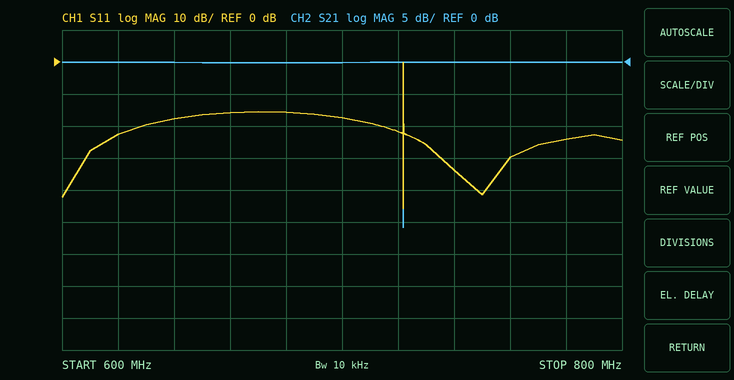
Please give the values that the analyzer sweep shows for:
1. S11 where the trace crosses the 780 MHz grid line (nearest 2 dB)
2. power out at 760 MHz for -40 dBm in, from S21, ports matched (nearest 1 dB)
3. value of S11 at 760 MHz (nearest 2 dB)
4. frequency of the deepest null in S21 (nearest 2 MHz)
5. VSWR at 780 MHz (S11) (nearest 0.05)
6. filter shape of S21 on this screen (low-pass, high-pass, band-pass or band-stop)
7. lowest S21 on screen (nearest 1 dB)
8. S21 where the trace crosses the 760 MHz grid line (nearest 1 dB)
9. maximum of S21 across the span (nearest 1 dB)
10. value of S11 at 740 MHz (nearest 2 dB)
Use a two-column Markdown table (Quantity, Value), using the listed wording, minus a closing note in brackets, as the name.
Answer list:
| Quantity | Value |
|---|---|
| S11 where the trace crosses the 780 MHz grid line | -24 dB |
| power out at 760 MHz for -40 dBm in, from S21, ports matched | -40 dBm |
| value of S11 at 760 MHz | -30 dB |
| frequency of the deepest null in S21 | 722 MHz |
| VSWR at 780 MHz (S11) | 1.15 |
| filter shape of S21 on this screen | band-stop |
| lowest S21 on screen | -26 dB |
| S21 where the trace crosses the 760 MHz grid line | 0 dB |
| maximum of S21 across the span | 0 dB |
| value of S11 at 740 MHz | -34 dB |
